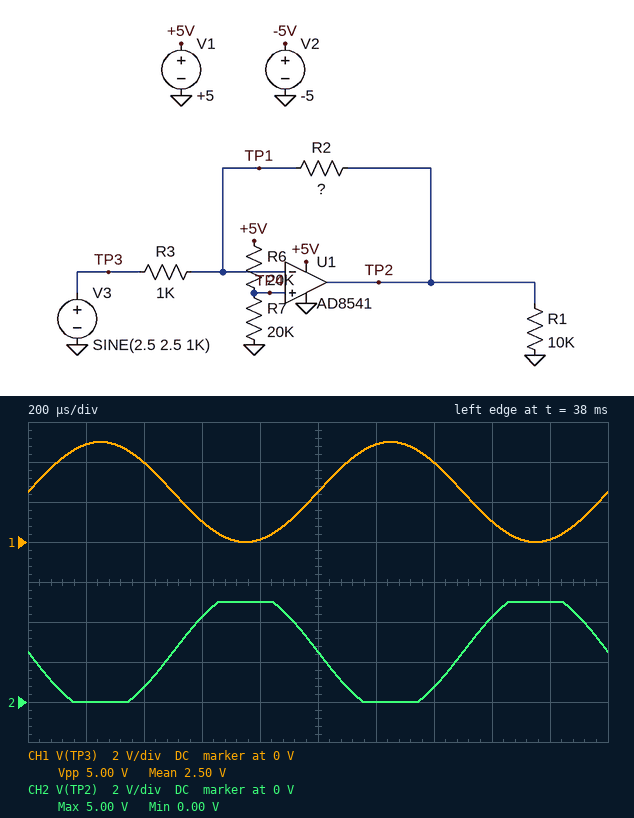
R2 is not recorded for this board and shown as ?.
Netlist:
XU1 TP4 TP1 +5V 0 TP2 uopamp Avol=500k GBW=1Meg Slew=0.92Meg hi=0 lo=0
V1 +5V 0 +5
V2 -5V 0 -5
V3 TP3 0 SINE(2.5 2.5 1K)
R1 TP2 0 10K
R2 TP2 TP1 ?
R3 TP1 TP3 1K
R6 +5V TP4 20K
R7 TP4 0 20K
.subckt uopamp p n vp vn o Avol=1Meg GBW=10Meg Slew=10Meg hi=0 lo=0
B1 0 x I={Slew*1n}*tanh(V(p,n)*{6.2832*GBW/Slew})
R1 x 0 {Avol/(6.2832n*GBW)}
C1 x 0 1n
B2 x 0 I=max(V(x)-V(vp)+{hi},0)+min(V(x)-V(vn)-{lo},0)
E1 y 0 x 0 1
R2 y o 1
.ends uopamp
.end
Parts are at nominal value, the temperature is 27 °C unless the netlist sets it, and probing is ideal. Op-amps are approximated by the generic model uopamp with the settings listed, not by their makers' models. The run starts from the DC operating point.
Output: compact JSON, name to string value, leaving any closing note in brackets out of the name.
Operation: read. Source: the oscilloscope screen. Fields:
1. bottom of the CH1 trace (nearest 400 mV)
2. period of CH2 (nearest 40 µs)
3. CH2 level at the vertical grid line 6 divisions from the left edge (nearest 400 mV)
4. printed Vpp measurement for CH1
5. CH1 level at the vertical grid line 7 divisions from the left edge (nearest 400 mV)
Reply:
{"bottom of the CH1 trace": "0 V", "period of CH2": "1.00 ms", "CH2 level at the vertical grid line 6 divisions from the left edge": "0 V", "printed Vpp measurement for CH1": "5.00 V", "CH1 level at the vertical grid line 7 divisions from the left edge": "4.0 V"}
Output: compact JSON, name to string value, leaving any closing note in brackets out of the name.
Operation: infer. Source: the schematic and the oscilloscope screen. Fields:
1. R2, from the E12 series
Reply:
{"R2, from the E12 series": "1.2 kΩ"}
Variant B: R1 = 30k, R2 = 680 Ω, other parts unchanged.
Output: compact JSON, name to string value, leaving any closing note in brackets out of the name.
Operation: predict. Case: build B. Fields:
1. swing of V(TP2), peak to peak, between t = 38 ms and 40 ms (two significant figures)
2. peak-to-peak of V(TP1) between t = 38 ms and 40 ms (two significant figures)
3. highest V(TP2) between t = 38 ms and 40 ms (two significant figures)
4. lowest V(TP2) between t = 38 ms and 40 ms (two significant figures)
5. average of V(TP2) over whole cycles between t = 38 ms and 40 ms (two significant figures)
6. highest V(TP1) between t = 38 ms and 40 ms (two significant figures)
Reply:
{"swing of V(TP2), peak to peak, between t = 38 ms and 40 ms": "3.4 V", "peak-to-peak of V(TP1) between t = 38 ms and 40 ms": "3.4 mV", "highest V(TP2) between t = 38 ms and 40 ms": "4.2 V", "lowest V(TP2) between t = 38 ms and 40 ms": "800 mV", "average of V(TP2) over whole cycles between t = 38 ms and 40 ms": "2.5 V", "highest V(TP1) between t = 38 ms and 40 ms": "2.5 V"}
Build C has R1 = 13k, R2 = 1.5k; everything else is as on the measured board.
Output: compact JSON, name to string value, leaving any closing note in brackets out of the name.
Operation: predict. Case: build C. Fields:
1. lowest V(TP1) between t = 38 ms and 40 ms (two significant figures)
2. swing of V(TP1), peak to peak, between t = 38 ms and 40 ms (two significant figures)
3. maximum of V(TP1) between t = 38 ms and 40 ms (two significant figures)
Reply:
{"lowest V(TP1) between t = 38 ms and 40 ms": "2.0 V", "swing of V(TP1), peak to peak, between t = 38 ms and 40 ms": "1.0 V", "maximum of V(TP1) between t = 38 ms and 40 ms": "3.0 V"}
